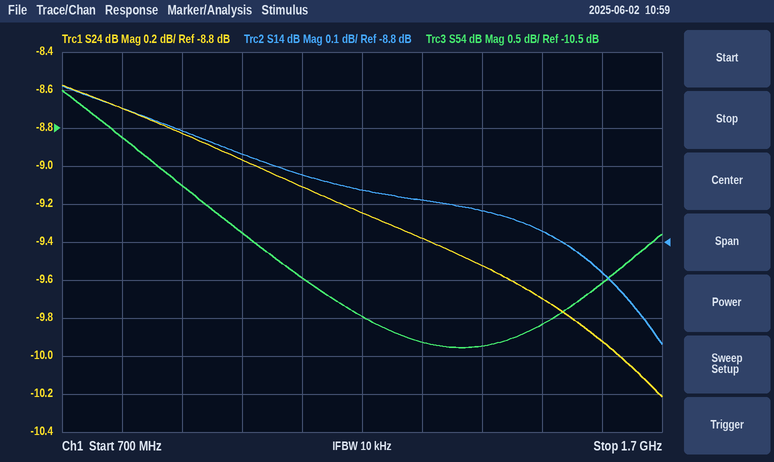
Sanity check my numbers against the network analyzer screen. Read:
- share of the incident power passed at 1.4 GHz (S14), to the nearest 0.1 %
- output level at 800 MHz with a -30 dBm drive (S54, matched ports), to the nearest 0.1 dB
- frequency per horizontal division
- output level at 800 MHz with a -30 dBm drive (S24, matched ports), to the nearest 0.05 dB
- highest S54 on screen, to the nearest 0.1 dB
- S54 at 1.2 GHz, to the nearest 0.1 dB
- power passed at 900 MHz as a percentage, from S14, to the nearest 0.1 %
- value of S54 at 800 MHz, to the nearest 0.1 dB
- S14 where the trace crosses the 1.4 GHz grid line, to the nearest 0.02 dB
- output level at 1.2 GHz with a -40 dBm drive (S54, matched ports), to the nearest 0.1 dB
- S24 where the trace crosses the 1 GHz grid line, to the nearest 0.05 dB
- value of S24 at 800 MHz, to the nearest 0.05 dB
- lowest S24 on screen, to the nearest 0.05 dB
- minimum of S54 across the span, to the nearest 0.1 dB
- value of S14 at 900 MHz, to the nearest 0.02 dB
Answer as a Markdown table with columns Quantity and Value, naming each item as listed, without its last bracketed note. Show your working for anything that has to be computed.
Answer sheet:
| Quantity | Value |
|---|---|
| share of the incident power passed at 1.4 GHz (S14), to the nearest 0.1 % | 10^(-8.72/10) ≈ 13.4 % |
| output level at 800 MHz with a -30 dBm drive (S54, matched ports), to the nearest 0.1 dB | -30 dBm + (-10.6 dB) = -40.6 dBm |
| frequency per horizontal division | 100 MHz |
| output level at 800 MHz with a -30 dBm drive (S24, matched ports), to the nearest 0.05 dB | -30 dBm + (-8.70 dB) = -38.70 dBm |
| highest S54 on screen, to the nearest 0.1 dB | -10.0 dB |
| S54 at 1.2 GHz, to the nearest 0.1 dB | -13.0 dB |
| power passed at 900 MHz as a percentage, from S14, to the nearest 0.1 % | 10^(-8.5/10) ≈ 14.1 % |
| value of S54 at 800 MHz, to the nearest 0.1 dB | -10.6 dB |
| S14 where the trace crosses the 1.4 GHz grid line, to the nearest 0.02 dB | -8.72 dB |
| output level at 1.2 GHz with a -40 dBm drive (S54, matched ports), to the nearest 0.1 dB | -40 dBm + (-13.0 dB) = -53.0 dBm |
| S24 where the trace crosses the 1 GHz grid line, to the nearest 0.05 dB | -8.95 dB |
| value of S24 at 800 MHz, to the nearest 0.05 dB | -8.70 dB |
| lowest S24 on screen, to the nearest 0.05 dB | -10.20 dB |
| minimum of S54 across the span, to the nearest 0.1 dB | -13.4 dB |
| value of S14 at 900 MHz, to the nearest 0.02 dB | -8.50 dB |
